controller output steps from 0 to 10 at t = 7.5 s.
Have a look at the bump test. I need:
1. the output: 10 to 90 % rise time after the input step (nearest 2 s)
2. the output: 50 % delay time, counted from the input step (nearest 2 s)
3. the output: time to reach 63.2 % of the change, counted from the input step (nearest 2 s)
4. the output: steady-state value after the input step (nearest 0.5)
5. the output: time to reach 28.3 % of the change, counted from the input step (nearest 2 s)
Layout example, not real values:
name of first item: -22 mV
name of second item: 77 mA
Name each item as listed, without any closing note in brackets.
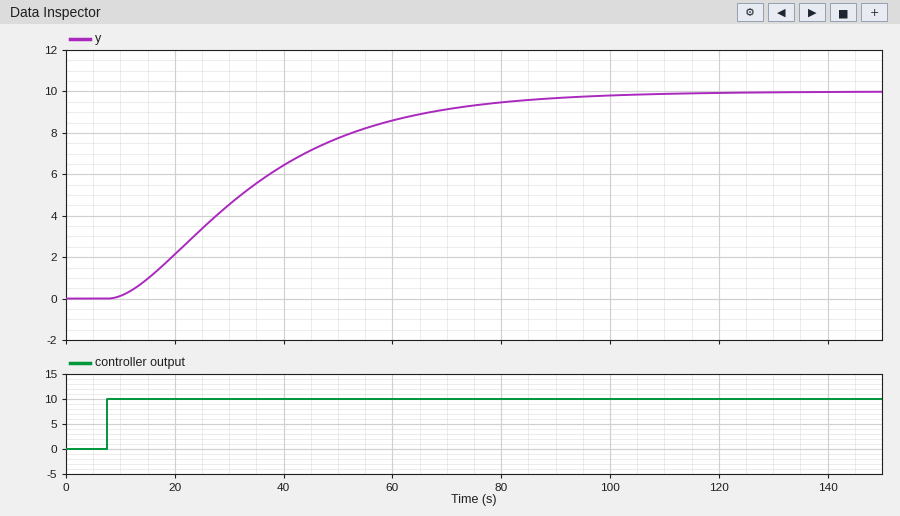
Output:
the output: 10 to 90 % rise time after the input step: 52 s
the output: 50 % delay time, counted from the input step: 24 s
the output: time to reach 63.2 % of the change, counted from the input step: 32 s
the output: steady-state value after the input step: 10.0
the output: time to reach 28.3 % of the change, counted from the input step: 16 s
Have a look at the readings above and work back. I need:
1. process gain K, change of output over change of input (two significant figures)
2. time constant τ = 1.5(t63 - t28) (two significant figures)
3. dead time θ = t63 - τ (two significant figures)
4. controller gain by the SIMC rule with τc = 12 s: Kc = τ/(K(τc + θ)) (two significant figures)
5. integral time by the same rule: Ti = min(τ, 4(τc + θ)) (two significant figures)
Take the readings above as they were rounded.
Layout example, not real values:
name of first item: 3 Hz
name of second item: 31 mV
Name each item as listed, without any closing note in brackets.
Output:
process gain K, change of output over change of input: 1.0
time constant τ = 1.5(t63 - t28): 24 s
dead time θ = t63 - τ: 8.0 s
controller gain by the SIMC rule with τc = 12 s: Kc = τ/(K(τc + θ)): 1.2
integral time by the same rule: Ti = min(τ, 4(τc + θ)): 24 s
